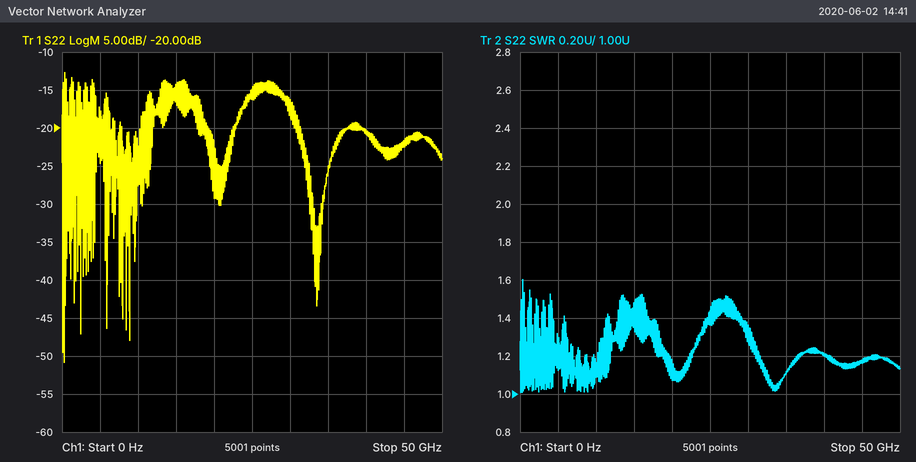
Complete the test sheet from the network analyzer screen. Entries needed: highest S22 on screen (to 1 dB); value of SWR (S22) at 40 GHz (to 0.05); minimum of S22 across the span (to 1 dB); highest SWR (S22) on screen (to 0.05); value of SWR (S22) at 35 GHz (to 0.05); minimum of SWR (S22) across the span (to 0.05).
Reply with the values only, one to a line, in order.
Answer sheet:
-13 dB
1.20
-51 dB
1.60
1.10
1.00
